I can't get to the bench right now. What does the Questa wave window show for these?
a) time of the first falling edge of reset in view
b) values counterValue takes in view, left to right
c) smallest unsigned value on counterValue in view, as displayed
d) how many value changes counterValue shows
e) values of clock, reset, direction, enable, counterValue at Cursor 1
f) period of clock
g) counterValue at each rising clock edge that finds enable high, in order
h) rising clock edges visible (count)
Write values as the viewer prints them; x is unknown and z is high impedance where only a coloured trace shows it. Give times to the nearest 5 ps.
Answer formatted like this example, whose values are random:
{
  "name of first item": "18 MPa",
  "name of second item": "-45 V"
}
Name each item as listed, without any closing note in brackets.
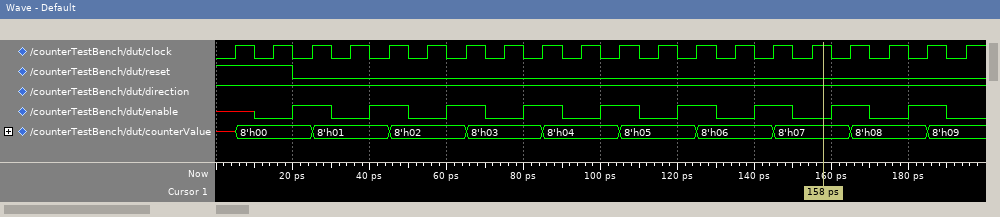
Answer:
{
  "time of the first falling edge of reset in view": "20 ps",
  "values counterValue takes in view, left to right": "x, 8'h00, 8'h01, 8'h02, 8'h03, 8'h04, 8'h05, 8'h06, 8'h07, 8'h08, 8'h09",
  "smallest unsigned value on counterValue in view, as displayed": "8'h00",
  "how many value changes counterValue shows": "10",
  "values of clock, reset, direction, enable, counterValue at Cursor 1": "clock=1, reset=0, direction=1, enable=0, counterValue=8'h07",
  "period of clock": "10 ps",
  "counterValue at each rising clock edge that finds enable high, in order": "8'h00, 8'h01, 8'h02, 8'h03, 8'h04, 8'h05, 8'h06, 8'h07, 8'h08",
  "rising clock edges visible": "20"
}
